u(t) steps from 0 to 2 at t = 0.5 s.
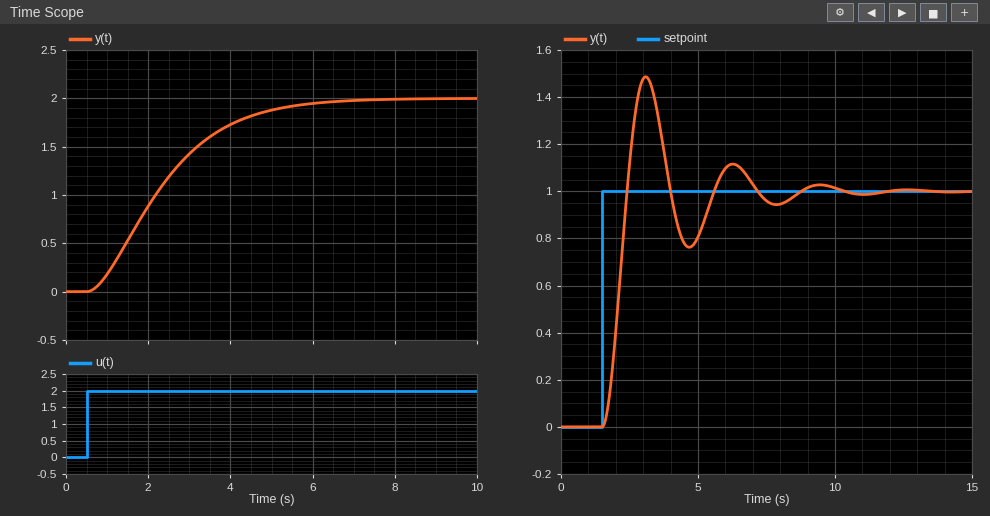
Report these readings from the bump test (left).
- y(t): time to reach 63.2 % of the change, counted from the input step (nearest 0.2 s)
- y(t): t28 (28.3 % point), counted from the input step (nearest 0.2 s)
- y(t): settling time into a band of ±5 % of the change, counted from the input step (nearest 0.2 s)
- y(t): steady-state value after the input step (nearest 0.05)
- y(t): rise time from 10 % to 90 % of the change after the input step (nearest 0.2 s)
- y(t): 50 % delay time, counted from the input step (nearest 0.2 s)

2.2 s
1.0 s
4.8 s
2.00
3.4 s
1.6 s
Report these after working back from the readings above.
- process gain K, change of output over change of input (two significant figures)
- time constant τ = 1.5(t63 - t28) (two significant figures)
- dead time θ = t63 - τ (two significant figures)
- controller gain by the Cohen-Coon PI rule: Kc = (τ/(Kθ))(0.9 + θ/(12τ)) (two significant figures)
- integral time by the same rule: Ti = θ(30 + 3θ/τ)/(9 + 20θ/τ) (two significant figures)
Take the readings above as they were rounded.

1.0
1.8 s
0.40 s
4.1
0.91 s
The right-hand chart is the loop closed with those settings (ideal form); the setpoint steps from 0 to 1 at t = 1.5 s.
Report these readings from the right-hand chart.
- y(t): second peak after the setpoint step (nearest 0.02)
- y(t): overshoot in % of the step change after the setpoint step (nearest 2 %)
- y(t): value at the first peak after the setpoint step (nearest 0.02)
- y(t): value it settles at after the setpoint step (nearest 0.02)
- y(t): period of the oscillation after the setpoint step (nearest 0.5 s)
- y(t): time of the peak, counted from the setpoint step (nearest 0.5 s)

1.12
48 %
1.48
1.00
3.0 s
1.5 s
